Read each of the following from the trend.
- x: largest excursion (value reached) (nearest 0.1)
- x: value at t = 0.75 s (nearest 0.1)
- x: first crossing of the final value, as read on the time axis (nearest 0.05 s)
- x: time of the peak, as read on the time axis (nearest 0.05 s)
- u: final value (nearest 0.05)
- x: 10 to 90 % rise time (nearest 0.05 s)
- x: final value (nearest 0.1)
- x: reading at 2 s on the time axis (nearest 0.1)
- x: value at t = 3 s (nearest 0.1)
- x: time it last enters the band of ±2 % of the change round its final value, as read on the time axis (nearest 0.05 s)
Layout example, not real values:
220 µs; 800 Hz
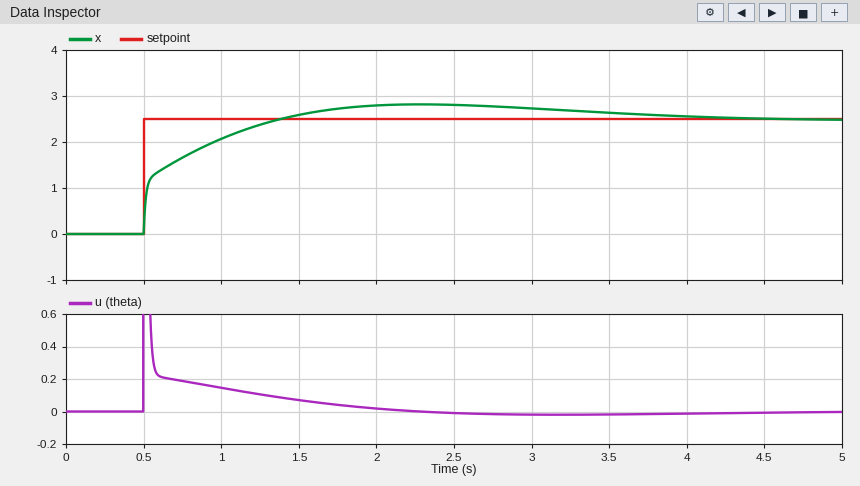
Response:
2.8; 1.7; 1.40 s; 2.30 s; 0.00; 0.65 s; 2.5; 2.8; 2.7; 4.05 s
